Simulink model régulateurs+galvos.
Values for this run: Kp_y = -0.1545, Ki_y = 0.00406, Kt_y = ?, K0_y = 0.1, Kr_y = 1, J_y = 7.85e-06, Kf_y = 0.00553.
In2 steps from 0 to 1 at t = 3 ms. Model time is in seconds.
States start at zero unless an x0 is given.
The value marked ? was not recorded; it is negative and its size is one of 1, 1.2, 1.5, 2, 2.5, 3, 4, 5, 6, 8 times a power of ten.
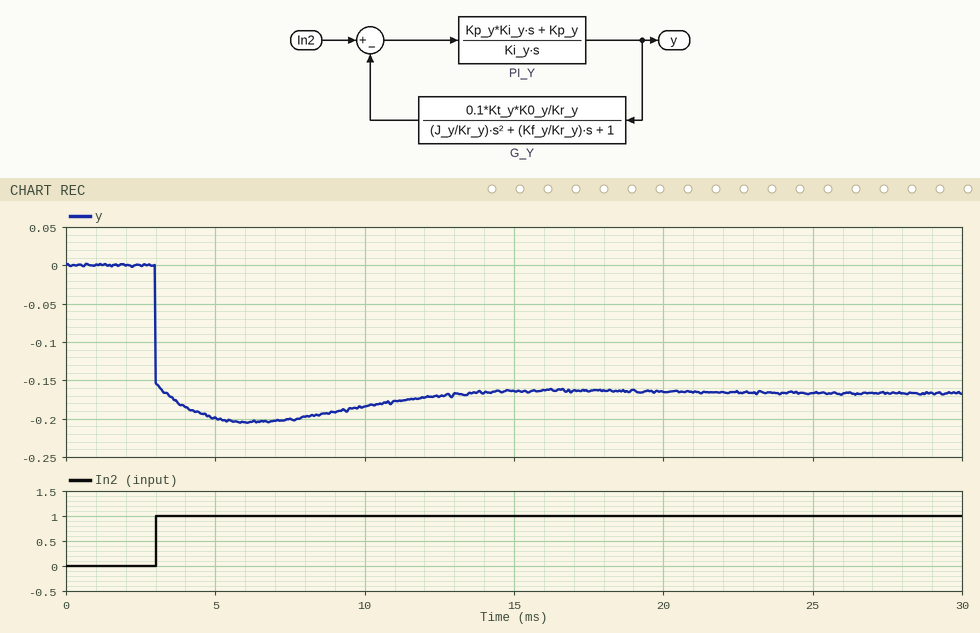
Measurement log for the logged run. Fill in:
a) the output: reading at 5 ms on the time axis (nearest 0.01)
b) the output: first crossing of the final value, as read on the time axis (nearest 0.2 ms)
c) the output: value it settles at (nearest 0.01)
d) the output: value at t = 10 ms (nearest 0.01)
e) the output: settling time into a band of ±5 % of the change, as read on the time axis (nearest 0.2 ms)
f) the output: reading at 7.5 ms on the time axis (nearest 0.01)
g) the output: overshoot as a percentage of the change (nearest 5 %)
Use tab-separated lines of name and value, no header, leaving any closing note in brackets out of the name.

the output: reading at 5 ms on the time axis	-0.20
the output: first crossing of the final value, as read on the time axis	3.4 ms
the output: value it settles at	-0.17
the output: value at t = 10 ms	-0.18
the output: settling time into a band of ±5 % of the change, as read on the time axis	11.4 ms
the output: reading at 7.5 ms on the time axis	-0.20
the output: overshoot as a percentage of the change	25 %
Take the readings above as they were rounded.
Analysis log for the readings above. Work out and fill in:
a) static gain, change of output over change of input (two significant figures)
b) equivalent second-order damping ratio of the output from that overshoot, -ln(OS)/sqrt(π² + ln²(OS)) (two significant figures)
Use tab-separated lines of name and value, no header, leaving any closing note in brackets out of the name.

static gain, change of output over change of input	-0.17
equivalent second-order damping ratio of the output from that overshoot, -ln(OS)/sqrt(π² + ln²(OS))	0.40
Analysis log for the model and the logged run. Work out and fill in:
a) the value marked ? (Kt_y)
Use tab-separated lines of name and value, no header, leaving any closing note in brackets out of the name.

the value marked ?	-600
